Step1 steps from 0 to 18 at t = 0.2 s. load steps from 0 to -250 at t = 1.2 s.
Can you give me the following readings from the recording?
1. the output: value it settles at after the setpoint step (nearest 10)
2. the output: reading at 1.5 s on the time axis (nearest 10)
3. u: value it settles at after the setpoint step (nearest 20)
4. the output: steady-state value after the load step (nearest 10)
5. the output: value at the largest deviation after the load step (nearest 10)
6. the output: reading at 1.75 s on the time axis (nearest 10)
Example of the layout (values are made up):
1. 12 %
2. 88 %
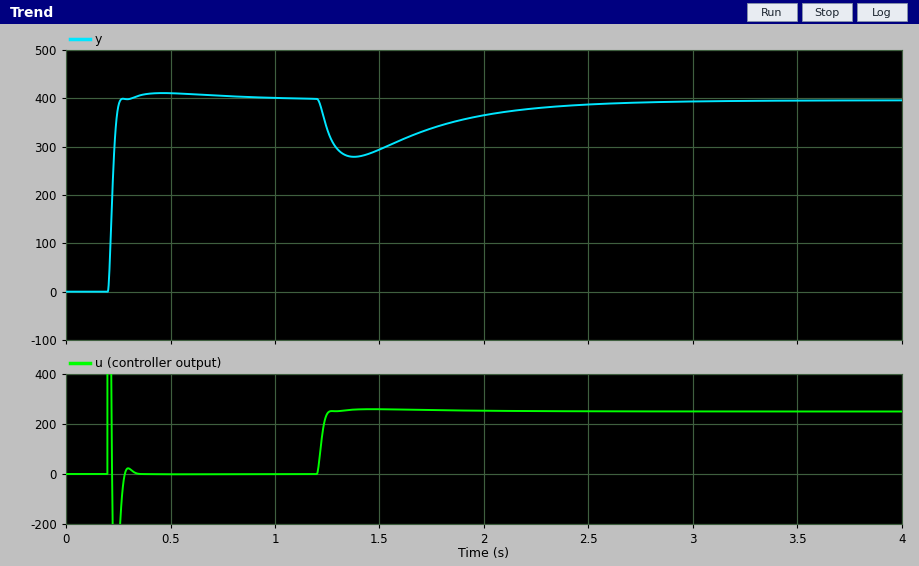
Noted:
1. 400
2. 290
3. 0
4. 400
5. 280
6. 340
